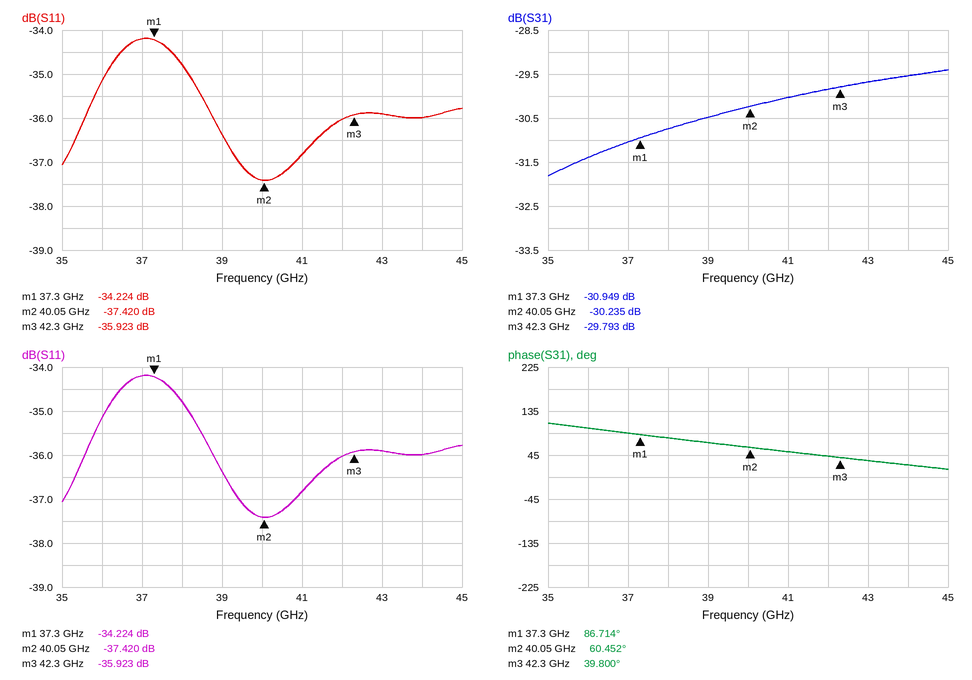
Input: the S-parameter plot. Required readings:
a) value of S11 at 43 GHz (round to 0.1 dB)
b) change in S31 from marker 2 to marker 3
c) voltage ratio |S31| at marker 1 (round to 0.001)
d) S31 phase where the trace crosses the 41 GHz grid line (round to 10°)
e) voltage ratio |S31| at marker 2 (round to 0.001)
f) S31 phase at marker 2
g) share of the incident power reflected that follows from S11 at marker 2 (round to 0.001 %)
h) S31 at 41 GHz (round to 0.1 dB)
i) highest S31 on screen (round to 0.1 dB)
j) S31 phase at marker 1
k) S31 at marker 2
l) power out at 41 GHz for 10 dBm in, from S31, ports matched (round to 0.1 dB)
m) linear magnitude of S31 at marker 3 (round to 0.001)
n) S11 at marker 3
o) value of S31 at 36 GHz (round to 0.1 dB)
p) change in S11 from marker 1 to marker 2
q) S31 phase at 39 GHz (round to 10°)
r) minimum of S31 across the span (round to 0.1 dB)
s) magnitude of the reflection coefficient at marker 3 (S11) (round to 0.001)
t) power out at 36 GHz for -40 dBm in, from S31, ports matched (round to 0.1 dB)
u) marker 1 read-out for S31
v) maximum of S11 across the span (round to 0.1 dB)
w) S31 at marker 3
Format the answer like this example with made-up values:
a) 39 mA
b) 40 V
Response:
a) -35.9 dB
b) 0.442 dB
c) 0.028
d) 50°
e) 0.031
f) 60.452°
g) 0.018 %
h) -30.0 dB
i) -29.4 dB
j) 86.714°
k) -30.235 dB
l) -20.0 dBm
m) 0.032
n) -35.923 dB
o) -31.4 dB
p) -3.196 dB
q) 70°
r) -31.8 dB
s) 0.016
t) -71.4 dBm
u) -30.949 dB
v) -34.2 dB
w) -29.793 dB
